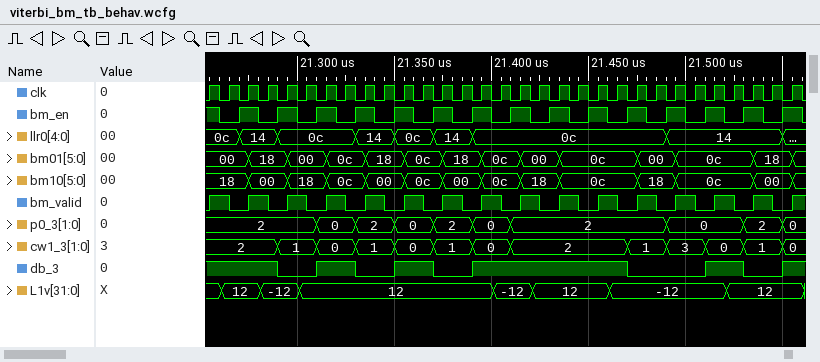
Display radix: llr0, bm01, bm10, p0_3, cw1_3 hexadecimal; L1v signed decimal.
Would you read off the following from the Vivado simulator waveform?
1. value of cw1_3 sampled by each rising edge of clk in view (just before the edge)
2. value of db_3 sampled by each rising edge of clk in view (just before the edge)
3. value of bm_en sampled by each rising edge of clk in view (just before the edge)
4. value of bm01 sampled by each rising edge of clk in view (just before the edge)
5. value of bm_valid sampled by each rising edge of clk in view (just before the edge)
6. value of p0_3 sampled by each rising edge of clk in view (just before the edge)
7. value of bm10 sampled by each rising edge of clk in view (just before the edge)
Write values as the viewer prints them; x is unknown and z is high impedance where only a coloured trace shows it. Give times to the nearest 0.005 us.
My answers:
2, 2, 2, 2, 1, 1, 0, 0, 1, 1, 0, 0, 1, 1, 0, 0, 2, 2, 2, 2, 2, 2, 1, 1, 3, 3, 0, 0, 1, 1, 0
1 1 1 1 0 0 1 1 0 0 1 1 0 0 1 1 1 1 1 1 1 1 0 0 0 0 1 1 0 0 1
1 0 1 0 1 0 1 0 1 0 1 0 1 0 1 0 1 0 1 0 1 0 1 0 1 0 1 0 1 0 1
00, 00, 00, 18, 18, 00, 00, 0c, 0c, 18, 18, 0c, 0c, 18, 18, 0c, 0c, 00, 00, 0c, 0c, 0c, 0c, 00, 00, 0c, 0c, 0c, 0c, 18, 18
0 1 0 1 0 1 0 1 0 1 0 1 0 1 0 1 0 1 0 1 0 1 0 1 0 1 0 1 0 1 0
2, 2, 2, 2, 2, 2, 0, 0, 2, 2, 0, 0, 2, 2, 0, 0, 2, 2, 2, 2, 2, 2, 2, 2, 0, 0, 0, 0, 2, 2, 0
18, 18, 18, 00, 00, 18, 18, 0c, 0c, 00, 00, 0c, 0c, 00, 00, 0c, 0c, 18, 18, 0c, 0c, 0c, 0c, 18, 18, 0c, 0c, 0c, 0c, 00, 00
